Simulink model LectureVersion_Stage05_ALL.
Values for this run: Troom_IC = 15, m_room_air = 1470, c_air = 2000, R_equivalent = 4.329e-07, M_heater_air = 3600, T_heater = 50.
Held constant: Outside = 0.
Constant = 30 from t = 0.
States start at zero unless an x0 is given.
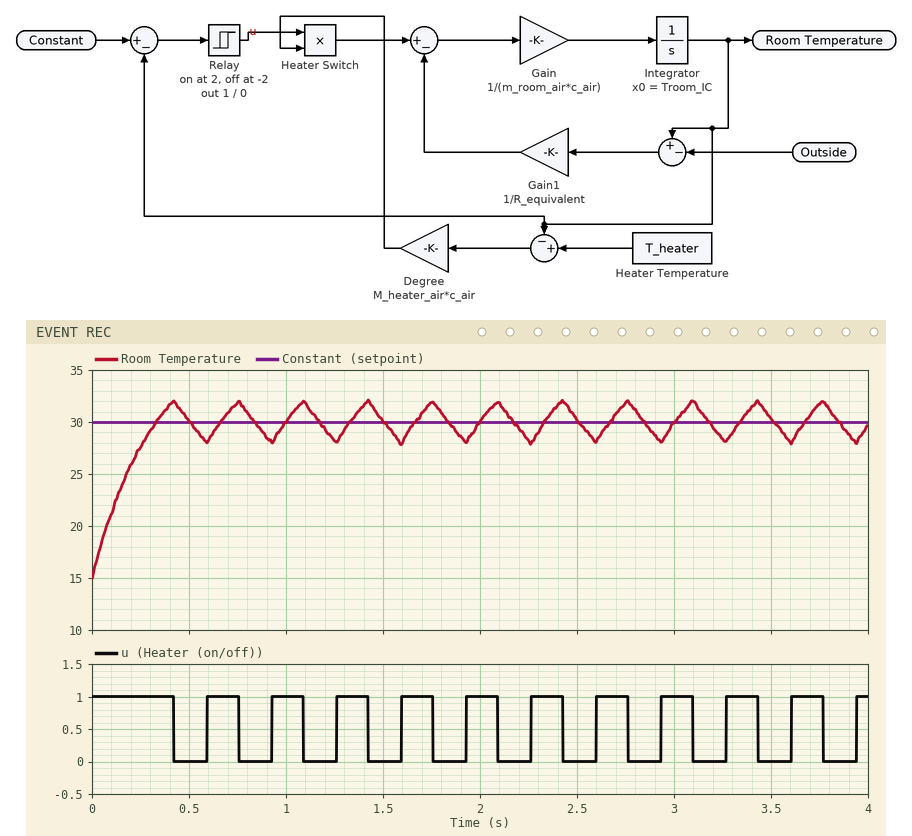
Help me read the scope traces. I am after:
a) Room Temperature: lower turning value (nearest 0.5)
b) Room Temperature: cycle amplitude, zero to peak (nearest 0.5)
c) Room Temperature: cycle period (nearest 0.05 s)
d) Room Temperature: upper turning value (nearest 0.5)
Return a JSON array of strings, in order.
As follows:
["28.0", "2.0", "0.35 s", "32.0"]
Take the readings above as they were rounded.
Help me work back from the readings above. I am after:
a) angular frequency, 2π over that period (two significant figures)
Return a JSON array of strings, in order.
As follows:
["18 rad/s"]
